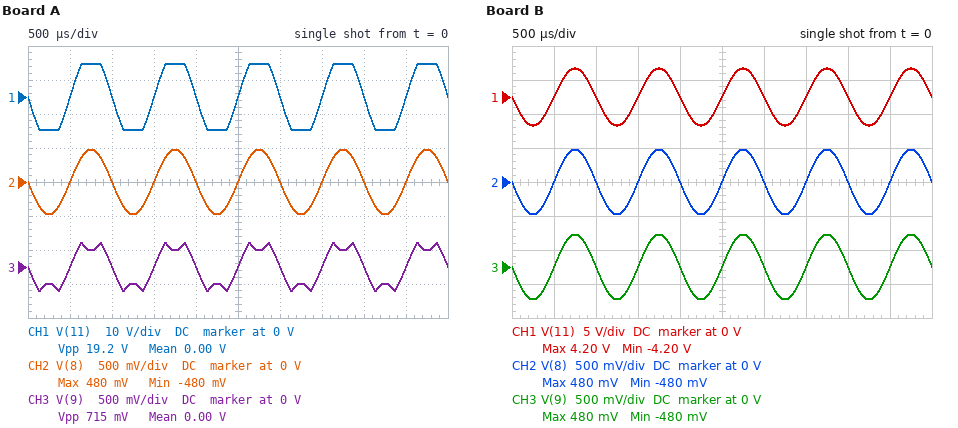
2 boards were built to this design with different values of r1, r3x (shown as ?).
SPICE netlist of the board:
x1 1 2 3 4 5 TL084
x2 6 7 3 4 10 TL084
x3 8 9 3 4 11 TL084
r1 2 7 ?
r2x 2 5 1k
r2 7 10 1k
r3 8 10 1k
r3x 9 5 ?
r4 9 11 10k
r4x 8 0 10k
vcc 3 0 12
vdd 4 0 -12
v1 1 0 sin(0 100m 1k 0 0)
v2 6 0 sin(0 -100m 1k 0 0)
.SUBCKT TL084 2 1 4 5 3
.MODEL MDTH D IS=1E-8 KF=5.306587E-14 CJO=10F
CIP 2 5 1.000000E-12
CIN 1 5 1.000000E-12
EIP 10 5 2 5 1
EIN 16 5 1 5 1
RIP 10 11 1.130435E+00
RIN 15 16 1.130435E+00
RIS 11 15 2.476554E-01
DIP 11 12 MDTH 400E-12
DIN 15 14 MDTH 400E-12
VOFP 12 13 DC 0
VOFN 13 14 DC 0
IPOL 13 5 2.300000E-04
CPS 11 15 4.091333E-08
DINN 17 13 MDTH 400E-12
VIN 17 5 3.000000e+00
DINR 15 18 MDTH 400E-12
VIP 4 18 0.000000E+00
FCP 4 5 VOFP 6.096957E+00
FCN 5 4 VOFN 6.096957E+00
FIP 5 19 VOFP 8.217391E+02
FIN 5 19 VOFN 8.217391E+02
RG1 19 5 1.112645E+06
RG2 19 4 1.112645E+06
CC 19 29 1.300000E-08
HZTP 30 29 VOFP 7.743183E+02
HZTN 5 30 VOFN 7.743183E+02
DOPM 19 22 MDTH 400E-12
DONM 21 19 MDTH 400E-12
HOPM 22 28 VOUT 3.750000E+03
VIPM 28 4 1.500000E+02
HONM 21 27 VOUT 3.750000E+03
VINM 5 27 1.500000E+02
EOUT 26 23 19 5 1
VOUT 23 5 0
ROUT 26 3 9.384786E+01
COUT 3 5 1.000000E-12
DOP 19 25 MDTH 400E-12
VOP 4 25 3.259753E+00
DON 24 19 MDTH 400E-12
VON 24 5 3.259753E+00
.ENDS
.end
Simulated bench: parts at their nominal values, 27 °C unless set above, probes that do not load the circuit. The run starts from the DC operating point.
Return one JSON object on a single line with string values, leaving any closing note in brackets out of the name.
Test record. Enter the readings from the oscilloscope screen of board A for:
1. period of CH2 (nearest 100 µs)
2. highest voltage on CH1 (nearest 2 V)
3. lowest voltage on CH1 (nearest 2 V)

{"period of CH2": "1.0 ms", "highest voltage on CH1": "10 V", "lowest voltage on CH1": "-10 V"}
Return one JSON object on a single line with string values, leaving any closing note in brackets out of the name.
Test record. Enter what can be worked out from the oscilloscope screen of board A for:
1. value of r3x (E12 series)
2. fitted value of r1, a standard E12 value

{"value of r3x": "820 Ω", "fitted value of r1, a standard E12 value": "470 Ω"}
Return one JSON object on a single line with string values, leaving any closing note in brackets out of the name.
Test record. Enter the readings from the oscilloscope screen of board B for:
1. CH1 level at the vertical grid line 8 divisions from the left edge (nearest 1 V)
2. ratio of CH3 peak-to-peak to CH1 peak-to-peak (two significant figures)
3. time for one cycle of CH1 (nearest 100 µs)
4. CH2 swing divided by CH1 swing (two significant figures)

{"CH1 level at the vertical grid line 8 divisions from the left edge": "0 V", "ratio of CH3 peak-to-peak to CH1 peak-to-peak": "0.11", "time for one cycle of CH1": "1.0 ms", "CH2 swing divided by CH1 swing": "0.11"}
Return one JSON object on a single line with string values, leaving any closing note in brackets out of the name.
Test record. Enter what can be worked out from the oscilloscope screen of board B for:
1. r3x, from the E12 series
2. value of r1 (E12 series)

{"r3x, from the E12 series": "2.7 kΩ", "value of r1": "470 Ω"}
